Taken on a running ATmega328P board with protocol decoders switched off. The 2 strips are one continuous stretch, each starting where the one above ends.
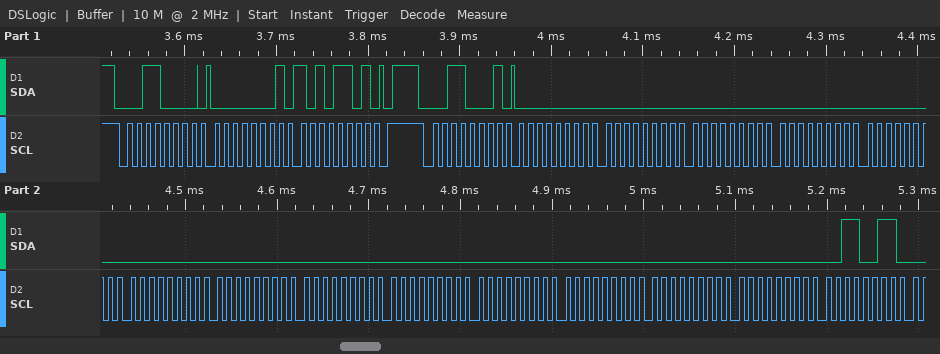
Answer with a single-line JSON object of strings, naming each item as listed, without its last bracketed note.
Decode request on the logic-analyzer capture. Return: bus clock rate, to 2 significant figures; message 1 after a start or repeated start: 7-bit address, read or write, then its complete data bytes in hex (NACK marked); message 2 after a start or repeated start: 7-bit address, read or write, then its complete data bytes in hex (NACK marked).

{"bus clock rate, to 2 significant figures": "100 kHz", "message 1 after a start or repeated start: 7-bit address, read or write, then its complete data bytes in hex": "0x18 write: 01 AD", "message 2 after a start or repeated start: 7-bit address, read or write, then its complete data bytes in hex": "0x18 read: 00 00 00 00 00 00 00 00 00 00 00 00 00 33"}
